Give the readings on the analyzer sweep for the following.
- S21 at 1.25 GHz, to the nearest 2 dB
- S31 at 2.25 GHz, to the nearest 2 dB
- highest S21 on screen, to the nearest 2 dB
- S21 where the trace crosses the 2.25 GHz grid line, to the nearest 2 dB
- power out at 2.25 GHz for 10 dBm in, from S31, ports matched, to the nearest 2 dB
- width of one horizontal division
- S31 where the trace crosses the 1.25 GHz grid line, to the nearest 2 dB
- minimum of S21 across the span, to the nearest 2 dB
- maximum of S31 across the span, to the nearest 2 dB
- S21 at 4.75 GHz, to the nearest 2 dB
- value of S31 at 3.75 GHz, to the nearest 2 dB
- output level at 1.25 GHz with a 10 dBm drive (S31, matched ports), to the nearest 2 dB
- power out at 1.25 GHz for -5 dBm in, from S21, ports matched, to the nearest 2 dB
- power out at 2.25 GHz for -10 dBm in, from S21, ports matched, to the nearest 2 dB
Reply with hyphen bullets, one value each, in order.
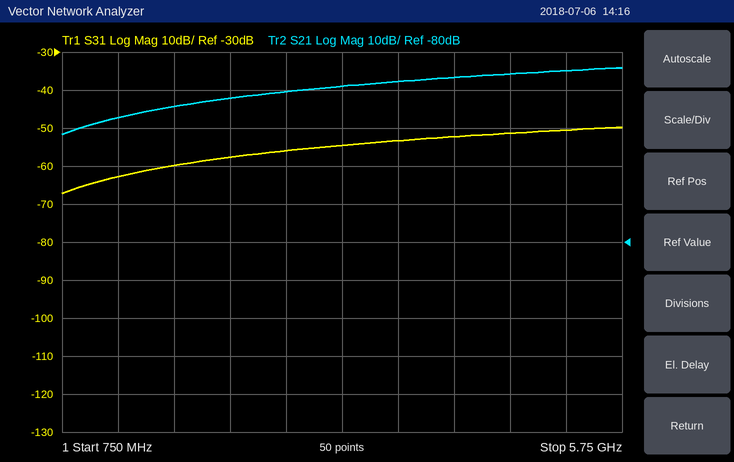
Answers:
- -48 dB
- -58 dB
- -34 dB
- -42 dB
- -48 dBm
- 500 MHz
- -62 dB
- -52 dB
- -50 dB
- -36 dB
- -54 dB
- -52 dBm
- -52 dBm
- -52 dBm
